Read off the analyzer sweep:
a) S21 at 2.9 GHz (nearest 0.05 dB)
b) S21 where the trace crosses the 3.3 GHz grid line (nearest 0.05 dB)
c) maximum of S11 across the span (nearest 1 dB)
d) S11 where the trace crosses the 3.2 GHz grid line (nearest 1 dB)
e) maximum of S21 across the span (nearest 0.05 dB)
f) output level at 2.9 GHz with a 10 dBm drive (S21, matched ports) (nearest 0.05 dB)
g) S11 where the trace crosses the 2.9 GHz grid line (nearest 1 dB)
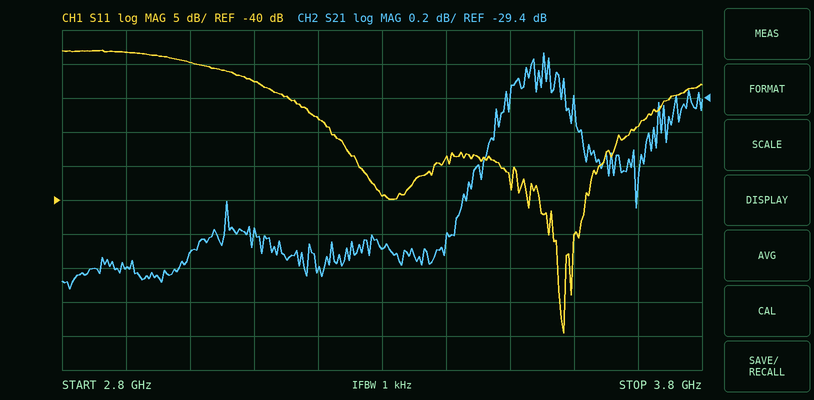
-30.40 dB
-30.30 dB
-18 dB
-28 dB
-29.15 dB
-20.40 dBm
-18 dB
